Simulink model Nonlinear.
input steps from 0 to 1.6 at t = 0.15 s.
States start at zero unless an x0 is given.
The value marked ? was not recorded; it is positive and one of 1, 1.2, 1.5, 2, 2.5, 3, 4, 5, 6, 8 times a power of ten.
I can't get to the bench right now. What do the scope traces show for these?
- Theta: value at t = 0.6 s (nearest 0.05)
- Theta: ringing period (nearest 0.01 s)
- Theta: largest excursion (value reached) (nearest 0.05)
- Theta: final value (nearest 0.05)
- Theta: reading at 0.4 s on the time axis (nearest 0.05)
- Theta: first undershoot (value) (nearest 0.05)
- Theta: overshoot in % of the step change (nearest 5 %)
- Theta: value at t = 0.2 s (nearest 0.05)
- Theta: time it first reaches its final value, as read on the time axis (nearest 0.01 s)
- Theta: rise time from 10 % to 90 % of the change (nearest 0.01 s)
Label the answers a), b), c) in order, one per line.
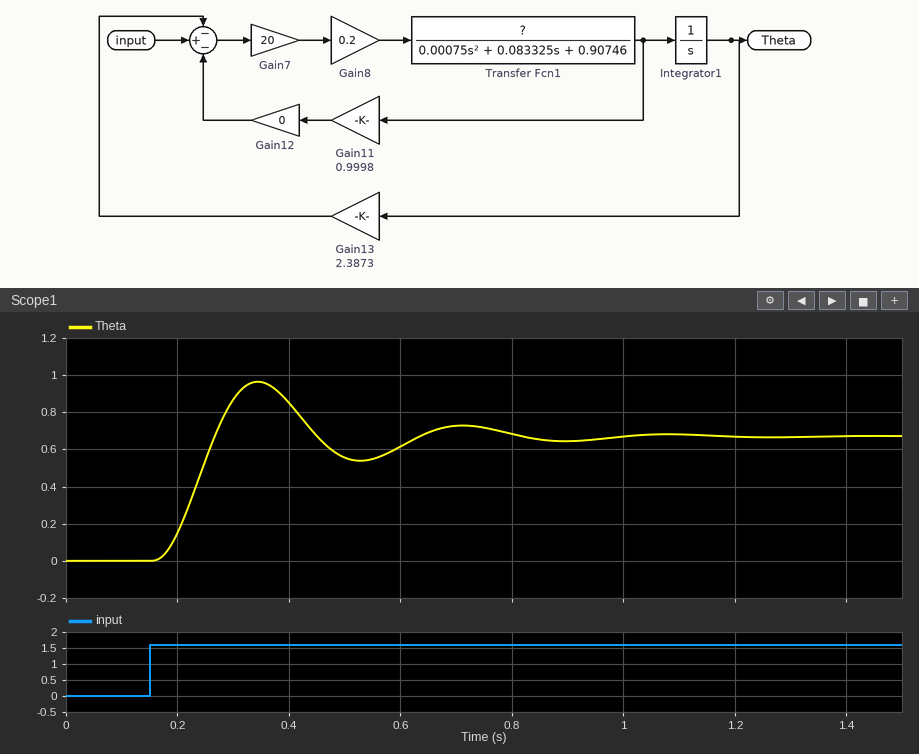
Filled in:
a) 0.60
b) 0.37 s
c) 0.95
d) 0.65
e) 0.85
f) 0.55
g) 45 %
h) 0.15
i) 0.27 s
j) 0.07 s
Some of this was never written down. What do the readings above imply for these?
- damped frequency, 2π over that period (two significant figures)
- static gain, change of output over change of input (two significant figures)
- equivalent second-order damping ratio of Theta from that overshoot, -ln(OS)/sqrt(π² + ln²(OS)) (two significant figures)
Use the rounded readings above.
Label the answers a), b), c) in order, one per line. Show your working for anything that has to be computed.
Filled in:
a) 2π / 0.37 = 17 rad/s
b) (0.65 - 0) / (1.6 - 0) = 0.41
c) ln(0.45) = -0.799; 0.799 / sqrt(9.870 + 0.638) = 0.25
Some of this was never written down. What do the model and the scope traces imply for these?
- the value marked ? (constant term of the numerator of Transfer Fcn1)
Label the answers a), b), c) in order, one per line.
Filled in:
a) 2.5
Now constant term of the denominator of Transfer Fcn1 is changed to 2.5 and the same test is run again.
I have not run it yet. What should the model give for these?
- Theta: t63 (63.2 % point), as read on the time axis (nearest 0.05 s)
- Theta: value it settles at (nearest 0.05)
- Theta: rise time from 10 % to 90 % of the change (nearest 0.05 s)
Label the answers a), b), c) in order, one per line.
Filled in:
a) 0.25 s
b) 0.65
c) 0.15 s
